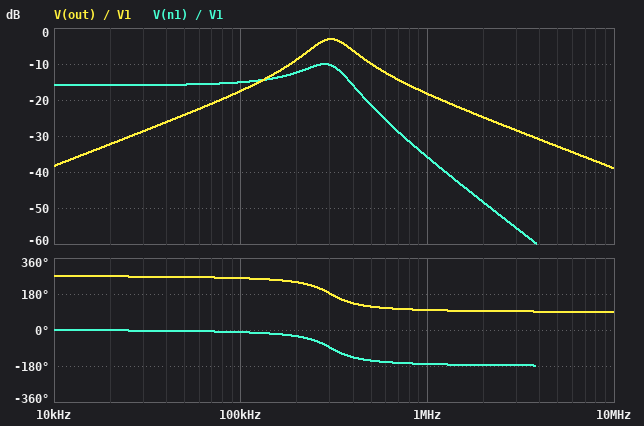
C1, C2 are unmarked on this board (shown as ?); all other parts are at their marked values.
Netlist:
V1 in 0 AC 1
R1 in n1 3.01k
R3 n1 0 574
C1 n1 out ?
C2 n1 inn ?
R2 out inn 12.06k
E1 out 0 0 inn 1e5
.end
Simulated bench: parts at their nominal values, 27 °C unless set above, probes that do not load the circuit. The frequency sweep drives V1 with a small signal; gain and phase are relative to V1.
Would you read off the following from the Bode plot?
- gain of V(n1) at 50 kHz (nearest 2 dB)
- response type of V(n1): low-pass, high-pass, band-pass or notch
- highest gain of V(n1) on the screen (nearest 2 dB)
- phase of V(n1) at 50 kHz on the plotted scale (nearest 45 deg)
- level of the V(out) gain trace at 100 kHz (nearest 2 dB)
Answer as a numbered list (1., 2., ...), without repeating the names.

1. -16 dB
2. low-pass
3. -10 dB
4. 0 deg
5. -18 dB
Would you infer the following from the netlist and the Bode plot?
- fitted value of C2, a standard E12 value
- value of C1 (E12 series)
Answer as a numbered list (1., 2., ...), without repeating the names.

1. 100 pF
2. 470 pF
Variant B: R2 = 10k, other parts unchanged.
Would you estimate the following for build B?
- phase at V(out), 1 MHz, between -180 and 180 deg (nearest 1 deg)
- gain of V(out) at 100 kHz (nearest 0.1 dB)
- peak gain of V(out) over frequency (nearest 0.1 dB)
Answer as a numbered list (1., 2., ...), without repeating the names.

1. 102 deg
2. -19.3 dB
3. -4.7 dB
